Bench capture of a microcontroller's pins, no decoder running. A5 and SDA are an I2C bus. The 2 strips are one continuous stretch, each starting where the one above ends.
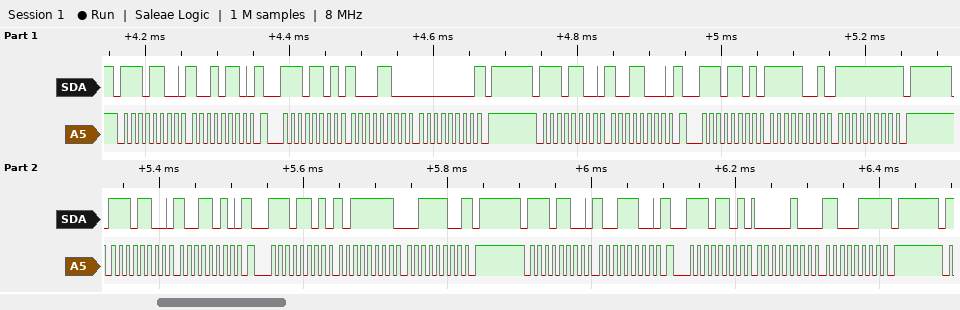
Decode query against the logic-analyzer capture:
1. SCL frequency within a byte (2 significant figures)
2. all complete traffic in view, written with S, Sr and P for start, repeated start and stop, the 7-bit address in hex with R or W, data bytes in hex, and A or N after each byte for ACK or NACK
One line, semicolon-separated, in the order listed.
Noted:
100 kHz; S 76W A 96 A Sr 76R A 8C A 00 N P S 76W A 98 A Sr 76R A F9 A FF N P S 76W A 9A A Sr 76R A BF A 3C N P S 76W A 9C A Sr 76R A 04 A C7 N P
